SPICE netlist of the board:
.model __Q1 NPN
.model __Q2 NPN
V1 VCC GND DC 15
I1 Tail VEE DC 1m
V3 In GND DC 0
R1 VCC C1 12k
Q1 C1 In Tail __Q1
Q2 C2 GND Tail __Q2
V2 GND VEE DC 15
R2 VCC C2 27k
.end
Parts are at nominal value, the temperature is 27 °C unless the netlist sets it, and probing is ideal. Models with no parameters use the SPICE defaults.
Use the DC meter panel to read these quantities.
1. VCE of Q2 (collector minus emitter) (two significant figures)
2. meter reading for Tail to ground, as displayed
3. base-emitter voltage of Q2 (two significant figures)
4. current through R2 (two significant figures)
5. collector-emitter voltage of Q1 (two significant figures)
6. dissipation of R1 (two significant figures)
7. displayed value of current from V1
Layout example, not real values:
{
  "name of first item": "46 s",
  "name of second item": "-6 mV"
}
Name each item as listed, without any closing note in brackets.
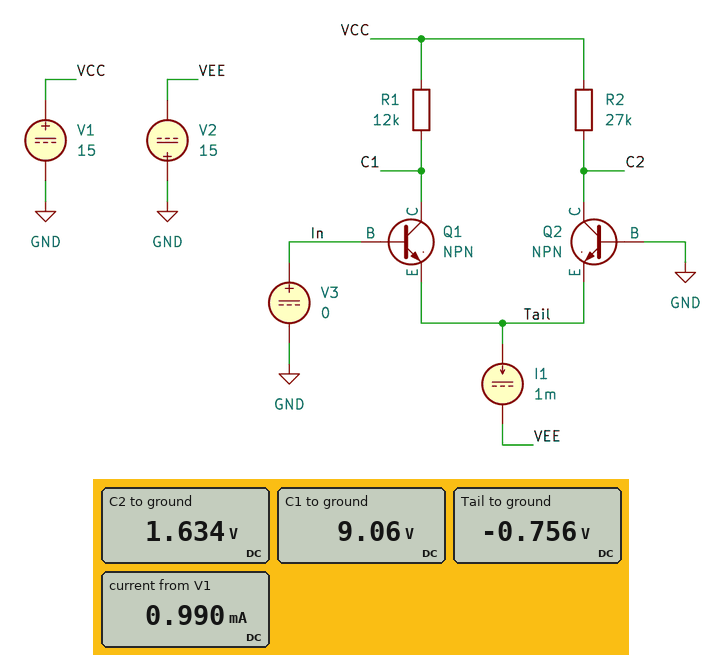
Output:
{
  "VCE of Q2 (collector minus emitter)": "2.4 V",
  "meter reading for Tail to ground, as displayed": "-0.756 V",
  "base-emitter voltage of Q2": "760 mV",
  "current through R2": "500 µA",
  "collector-emitter voltage of Q1": "9.8 V",
  "dissipation of R1": "2.9 mW",
  "displayed value of current from V1": "0.990 mA"
}
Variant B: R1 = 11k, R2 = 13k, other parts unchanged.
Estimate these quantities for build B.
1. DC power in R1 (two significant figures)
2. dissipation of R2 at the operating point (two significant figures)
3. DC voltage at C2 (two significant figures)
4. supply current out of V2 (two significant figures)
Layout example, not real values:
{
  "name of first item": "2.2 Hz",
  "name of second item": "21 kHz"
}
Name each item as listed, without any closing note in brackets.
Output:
{
  "DC power in R1": "2.7 mW",
  "dissipation of R2 at the operating point": "3.2 mW",
  "DC voltage at C2": "8.6 V",
  "supply current out of V2": "1.0 mA"
}
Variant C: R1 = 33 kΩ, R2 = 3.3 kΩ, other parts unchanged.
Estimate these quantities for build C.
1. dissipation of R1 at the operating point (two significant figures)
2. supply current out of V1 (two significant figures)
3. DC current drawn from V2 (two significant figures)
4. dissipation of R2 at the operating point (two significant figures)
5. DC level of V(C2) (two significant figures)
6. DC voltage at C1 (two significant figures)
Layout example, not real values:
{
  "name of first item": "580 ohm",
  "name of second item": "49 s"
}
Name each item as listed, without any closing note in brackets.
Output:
{
  "dissipation of R1 at the operating point": "7.4 mW",
  "supply current out of V1": "980 µA",
  "DC current drawn from V2": "1.0 mA",
  "dissipation of R2 at the operating point": "830 µW",
  "DC level of V(C2)": "13 V",
  "DC voltage at C1": "-660 mV"
}
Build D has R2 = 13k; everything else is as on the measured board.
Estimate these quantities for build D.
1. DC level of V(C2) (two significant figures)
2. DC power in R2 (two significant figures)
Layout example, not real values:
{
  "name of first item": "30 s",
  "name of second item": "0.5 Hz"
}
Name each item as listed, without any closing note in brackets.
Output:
{
  "DC level of V(C2)": "8.6 V",
  "DC power in R2": "3.2 mW"
}
